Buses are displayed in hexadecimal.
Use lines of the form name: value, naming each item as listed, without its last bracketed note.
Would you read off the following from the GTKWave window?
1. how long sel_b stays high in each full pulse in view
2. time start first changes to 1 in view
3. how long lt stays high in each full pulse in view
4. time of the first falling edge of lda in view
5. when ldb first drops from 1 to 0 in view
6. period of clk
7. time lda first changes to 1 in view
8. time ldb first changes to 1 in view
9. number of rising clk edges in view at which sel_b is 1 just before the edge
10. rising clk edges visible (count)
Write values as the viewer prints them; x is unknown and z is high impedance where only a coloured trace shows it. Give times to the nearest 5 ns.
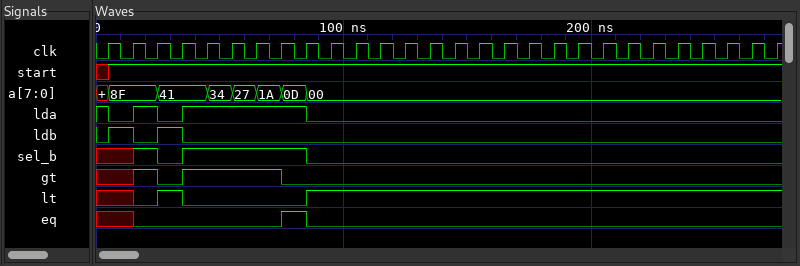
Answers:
how long sel_b stays high in each full pulse in view: 50 ns
time start first changes to 1 in view: 5 ns
how long lt stays high in each full pulse in view: 10 ns
time of the first falling edge of lda in view: 5 ns
when ldb first drops from 1 to 0 in view: 15 ns
period of clk: 10 ns
time lda first changes to 1 in view: 15 ns
time ldb first changes to 1 in view: 5 ns
number of rising clk edges in view at which sel_b is 1 just before the edge: 6
rising clk edges visible: 28
